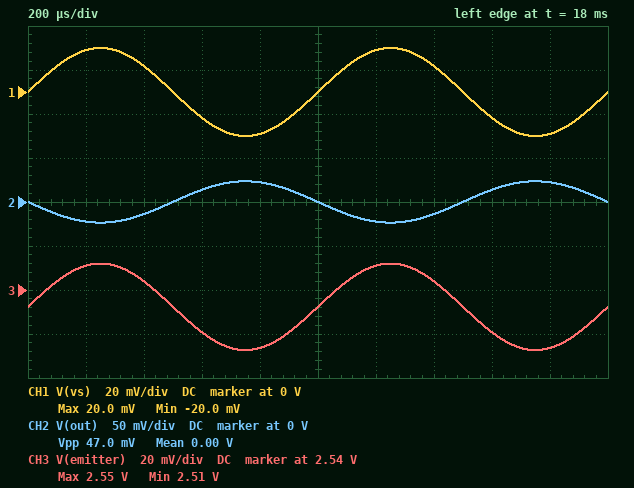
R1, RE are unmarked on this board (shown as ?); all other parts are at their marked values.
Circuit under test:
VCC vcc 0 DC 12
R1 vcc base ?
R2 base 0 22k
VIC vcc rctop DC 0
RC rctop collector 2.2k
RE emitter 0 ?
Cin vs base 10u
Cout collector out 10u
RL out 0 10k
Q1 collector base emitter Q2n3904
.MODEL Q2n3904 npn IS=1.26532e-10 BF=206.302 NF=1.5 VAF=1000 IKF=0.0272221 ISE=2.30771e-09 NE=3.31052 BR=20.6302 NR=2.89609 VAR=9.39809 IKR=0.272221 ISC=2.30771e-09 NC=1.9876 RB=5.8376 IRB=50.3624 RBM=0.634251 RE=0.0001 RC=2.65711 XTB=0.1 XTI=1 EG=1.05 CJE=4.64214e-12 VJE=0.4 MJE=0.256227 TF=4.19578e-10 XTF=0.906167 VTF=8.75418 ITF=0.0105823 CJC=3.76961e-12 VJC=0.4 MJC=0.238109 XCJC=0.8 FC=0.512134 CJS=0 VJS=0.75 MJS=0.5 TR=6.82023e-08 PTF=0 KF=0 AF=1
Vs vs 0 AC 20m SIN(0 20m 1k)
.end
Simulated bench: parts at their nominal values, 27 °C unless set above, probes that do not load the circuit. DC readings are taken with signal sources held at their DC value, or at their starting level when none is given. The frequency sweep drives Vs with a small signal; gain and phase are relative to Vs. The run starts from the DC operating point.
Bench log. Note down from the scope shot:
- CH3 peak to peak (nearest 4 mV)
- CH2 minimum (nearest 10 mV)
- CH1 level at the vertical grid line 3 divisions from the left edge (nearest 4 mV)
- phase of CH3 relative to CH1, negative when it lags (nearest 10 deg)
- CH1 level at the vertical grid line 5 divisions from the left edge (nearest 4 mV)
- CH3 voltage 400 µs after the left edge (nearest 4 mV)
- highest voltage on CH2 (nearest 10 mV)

40 mV
-20 mV
-12 mV
0 deg
0 V
2.544 V
20 mV
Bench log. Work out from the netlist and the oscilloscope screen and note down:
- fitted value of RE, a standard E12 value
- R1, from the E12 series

1.5 kΩ
56 kΩ
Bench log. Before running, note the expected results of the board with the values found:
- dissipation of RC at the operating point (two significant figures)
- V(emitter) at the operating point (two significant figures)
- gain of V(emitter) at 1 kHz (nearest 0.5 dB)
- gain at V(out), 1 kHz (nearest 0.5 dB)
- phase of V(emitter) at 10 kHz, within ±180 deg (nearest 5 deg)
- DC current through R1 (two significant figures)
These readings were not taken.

6.2 mW
2.5 V
0 dB
1.5 dB
0 deg
160 µA
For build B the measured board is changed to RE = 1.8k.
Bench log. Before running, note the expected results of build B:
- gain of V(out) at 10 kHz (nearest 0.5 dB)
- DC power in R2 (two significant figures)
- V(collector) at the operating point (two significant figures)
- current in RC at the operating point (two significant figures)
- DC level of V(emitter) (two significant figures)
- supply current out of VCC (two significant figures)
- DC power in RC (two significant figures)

0 dB
470 µW
8.9 V
1.4 mA
2.6 V
1.6 mA
4.4 mW
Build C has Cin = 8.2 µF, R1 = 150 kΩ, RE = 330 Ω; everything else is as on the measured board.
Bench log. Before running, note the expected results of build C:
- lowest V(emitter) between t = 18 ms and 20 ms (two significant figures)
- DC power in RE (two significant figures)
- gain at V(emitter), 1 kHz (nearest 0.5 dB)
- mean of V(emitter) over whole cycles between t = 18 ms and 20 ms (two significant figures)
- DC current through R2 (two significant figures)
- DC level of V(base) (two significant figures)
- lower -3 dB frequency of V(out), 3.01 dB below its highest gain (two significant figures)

590 mV
1.1 mW
-0.5 dB
610 mV
57 µA
1.3 V
2.1 Hz
